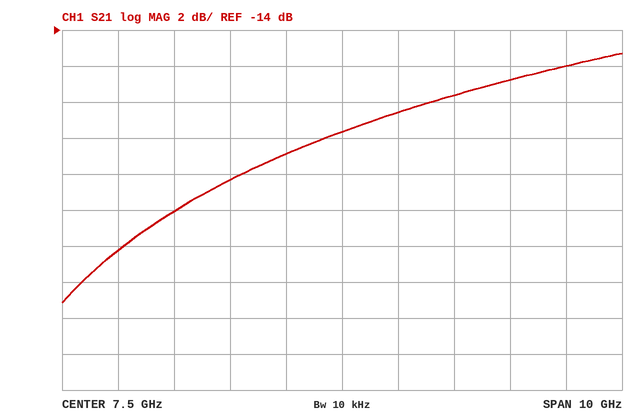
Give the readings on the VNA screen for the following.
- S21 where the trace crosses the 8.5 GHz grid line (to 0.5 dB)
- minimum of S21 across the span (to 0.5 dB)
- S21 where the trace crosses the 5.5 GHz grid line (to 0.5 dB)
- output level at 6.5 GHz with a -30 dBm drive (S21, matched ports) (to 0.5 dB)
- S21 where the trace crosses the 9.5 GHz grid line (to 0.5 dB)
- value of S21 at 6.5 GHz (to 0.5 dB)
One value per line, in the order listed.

-18.5 dB
-29.0 dB
-22.5 dB
-51.0 dBm
-17.5 dB
-21.0 dB
